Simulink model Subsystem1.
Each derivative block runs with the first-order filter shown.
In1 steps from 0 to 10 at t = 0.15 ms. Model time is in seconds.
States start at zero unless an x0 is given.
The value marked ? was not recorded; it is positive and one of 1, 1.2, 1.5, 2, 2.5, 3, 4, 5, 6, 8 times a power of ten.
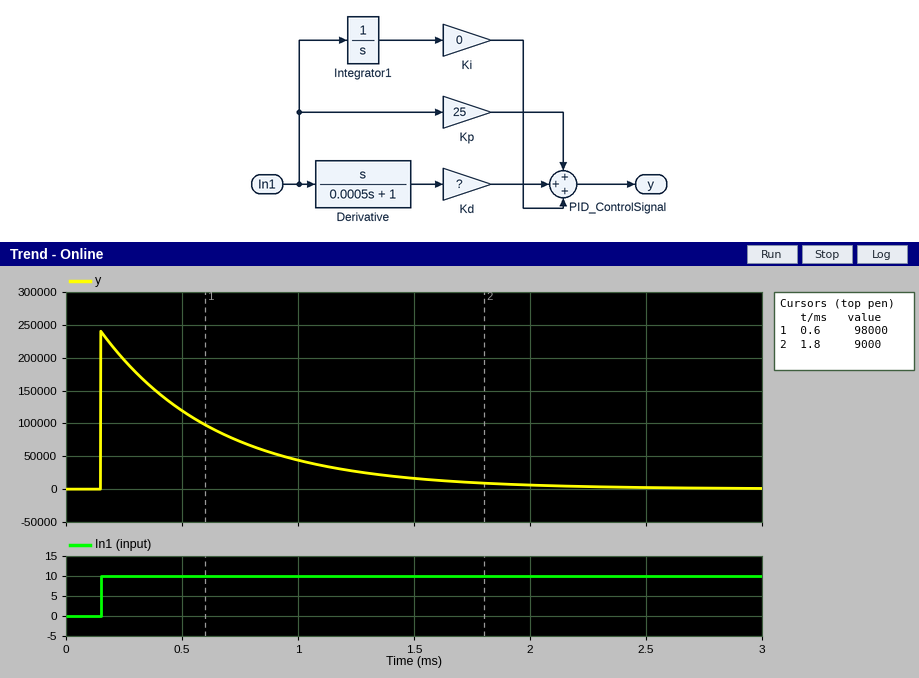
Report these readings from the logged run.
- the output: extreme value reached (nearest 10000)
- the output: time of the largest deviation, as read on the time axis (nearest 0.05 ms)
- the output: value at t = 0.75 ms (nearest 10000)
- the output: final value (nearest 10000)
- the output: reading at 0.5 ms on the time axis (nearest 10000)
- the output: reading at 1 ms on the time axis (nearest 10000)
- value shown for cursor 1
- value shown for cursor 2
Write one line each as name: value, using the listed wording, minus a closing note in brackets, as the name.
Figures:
the output: extreme value reached: 240000
the output: time of the largest deviation, as read on the time axis: 0.15 ms
the output: value at t = 0.75 ms: 70000
the output: final value: 0
the output: reading at 0.5 ms on the time axis: 120000
the output: reading at 1 ms on the time axis: 40000
value shown for cursor 1: 98000
value shown for cursor 2: 9000
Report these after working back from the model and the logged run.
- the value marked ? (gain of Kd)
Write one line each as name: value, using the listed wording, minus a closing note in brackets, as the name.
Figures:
the value marked ?: 12
